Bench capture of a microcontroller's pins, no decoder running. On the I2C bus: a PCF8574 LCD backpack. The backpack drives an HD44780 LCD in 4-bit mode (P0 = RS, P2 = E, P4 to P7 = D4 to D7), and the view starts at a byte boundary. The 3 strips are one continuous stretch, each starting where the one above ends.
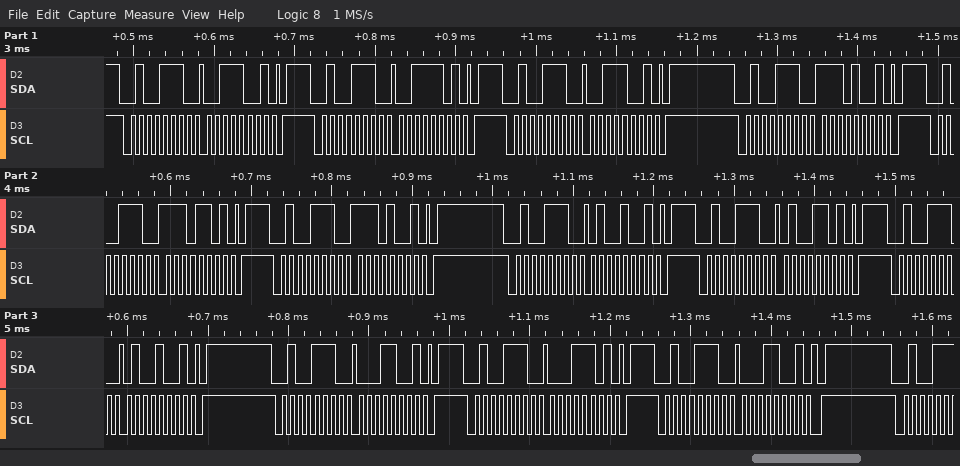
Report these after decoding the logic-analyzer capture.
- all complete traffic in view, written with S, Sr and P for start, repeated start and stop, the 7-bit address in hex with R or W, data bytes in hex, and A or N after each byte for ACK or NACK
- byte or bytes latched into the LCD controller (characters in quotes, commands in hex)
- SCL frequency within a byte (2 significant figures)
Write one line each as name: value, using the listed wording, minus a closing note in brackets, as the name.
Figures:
all complete traffic in view, written with S, Sr and P for start, repeated start and stop, the 7-bit address in hex with R or W, data bytes in hex, and A or N after each byte for ACK or NACK: S 27W A 39 A P S 27W A 3D A P S 27W A 39 A P S 27W A E9 A P S 27W A ED A P S 27W A E9 A P S 27W A 49 A P S 27W A 4D A P S 27W A 49 A P S 27W A 19 A P S 27W A 1D A P S 27W A 19 A P
byte or bytes latched into the LCD controller: '>' 'A'
SCL frequency within a byte: 100 kHz
